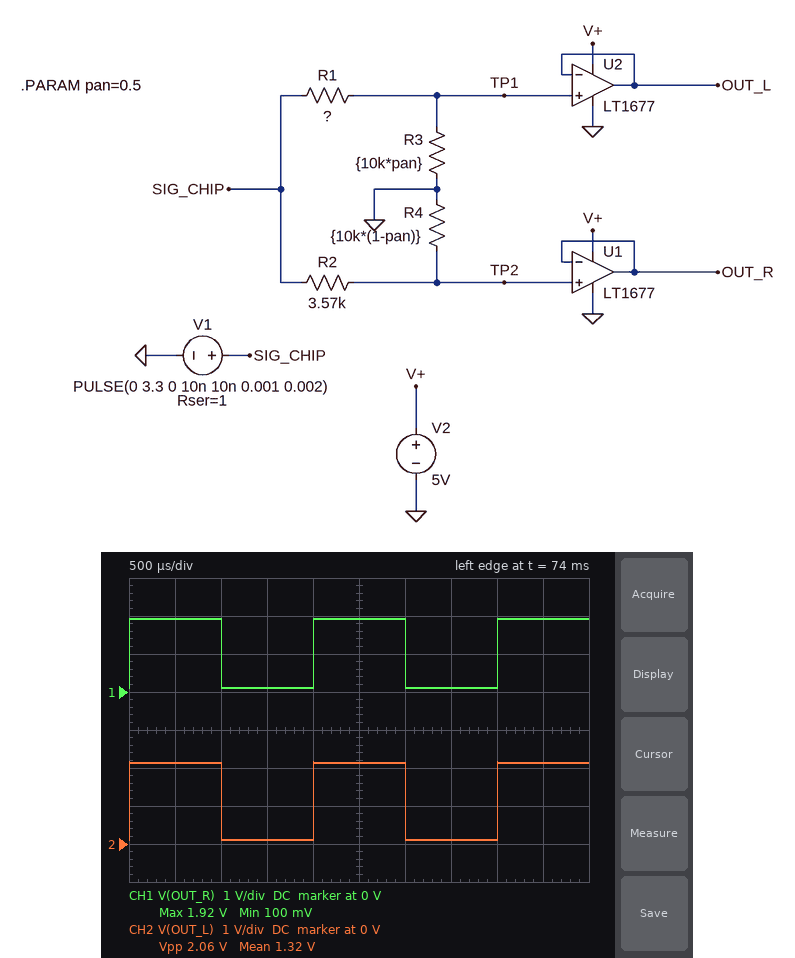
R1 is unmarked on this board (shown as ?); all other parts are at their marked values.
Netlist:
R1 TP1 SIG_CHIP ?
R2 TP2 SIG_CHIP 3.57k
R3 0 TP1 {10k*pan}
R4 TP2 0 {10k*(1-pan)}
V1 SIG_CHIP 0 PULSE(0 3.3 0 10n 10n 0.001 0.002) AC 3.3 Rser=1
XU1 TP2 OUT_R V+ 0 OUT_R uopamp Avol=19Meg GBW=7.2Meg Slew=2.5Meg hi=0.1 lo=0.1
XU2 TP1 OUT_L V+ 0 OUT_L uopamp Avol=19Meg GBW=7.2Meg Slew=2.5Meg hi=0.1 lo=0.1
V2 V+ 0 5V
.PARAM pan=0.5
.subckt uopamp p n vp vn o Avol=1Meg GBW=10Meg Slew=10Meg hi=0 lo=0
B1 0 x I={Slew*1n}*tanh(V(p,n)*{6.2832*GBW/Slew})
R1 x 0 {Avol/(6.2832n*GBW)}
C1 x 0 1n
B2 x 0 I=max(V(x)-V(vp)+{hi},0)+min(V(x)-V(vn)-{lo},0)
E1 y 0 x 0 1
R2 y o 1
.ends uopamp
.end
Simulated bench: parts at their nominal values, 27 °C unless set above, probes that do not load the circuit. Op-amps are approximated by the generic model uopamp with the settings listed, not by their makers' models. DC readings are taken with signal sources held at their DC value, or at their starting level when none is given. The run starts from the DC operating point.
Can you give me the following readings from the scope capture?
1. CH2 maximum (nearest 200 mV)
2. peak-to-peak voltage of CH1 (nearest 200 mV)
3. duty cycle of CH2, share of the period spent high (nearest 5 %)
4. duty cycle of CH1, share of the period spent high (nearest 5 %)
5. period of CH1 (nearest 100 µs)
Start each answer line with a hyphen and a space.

- 2.2 V
- 1.8 V
- 50 %
- 50 %
- 2.0 ms
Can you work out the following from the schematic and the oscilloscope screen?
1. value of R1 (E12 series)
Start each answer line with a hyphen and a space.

- 2.7 kΩ
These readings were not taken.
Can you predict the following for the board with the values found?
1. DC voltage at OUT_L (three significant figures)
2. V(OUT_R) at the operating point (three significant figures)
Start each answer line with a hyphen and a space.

- 97.6 mV
- 97.6 mV
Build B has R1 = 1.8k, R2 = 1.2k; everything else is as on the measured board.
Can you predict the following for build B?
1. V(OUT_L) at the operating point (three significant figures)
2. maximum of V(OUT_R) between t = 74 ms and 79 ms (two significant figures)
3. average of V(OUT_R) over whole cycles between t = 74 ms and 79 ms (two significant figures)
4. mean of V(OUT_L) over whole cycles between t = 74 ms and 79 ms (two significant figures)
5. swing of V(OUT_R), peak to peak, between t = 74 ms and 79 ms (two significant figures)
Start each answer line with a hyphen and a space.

- 97.6 mV
- 2.7 V
- 1.4 V
- 1.3 V
- 2.6 V
